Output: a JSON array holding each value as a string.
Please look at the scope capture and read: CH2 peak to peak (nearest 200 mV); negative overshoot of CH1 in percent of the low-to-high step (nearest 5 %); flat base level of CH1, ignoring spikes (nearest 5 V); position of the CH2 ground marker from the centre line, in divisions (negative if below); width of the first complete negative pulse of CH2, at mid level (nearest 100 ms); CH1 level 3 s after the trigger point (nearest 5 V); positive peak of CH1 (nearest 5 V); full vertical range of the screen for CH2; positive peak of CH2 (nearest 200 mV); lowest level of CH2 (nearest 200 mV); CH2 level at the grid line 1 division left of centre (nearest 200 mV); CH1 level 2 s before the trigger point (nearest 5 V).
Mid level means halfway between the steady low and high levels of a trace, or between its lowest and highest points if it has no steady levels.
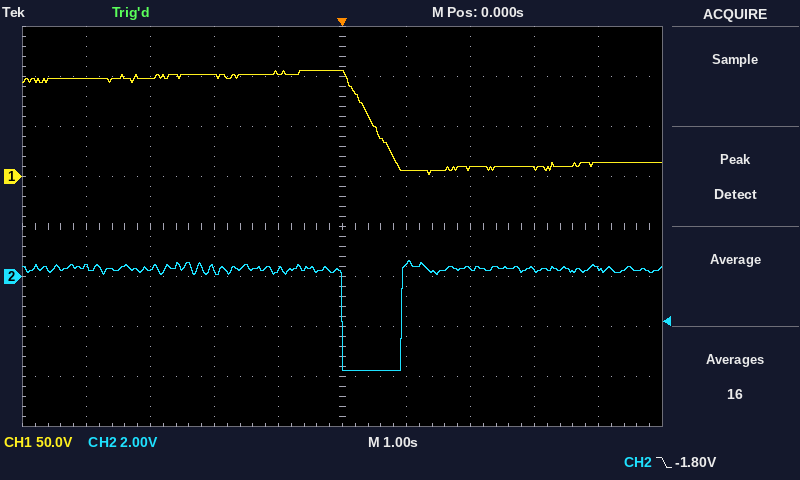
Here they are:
["4.4 V", "10 %", "10 V", "-1.0 div", "900 ms", "10 V", "105 V", "16 V", "600 mV", "-3.8 V", "200 mV", "100 V"]
